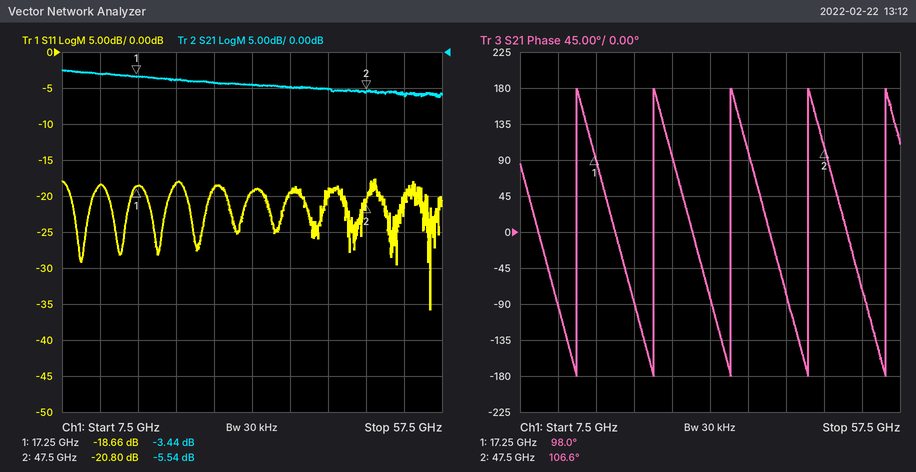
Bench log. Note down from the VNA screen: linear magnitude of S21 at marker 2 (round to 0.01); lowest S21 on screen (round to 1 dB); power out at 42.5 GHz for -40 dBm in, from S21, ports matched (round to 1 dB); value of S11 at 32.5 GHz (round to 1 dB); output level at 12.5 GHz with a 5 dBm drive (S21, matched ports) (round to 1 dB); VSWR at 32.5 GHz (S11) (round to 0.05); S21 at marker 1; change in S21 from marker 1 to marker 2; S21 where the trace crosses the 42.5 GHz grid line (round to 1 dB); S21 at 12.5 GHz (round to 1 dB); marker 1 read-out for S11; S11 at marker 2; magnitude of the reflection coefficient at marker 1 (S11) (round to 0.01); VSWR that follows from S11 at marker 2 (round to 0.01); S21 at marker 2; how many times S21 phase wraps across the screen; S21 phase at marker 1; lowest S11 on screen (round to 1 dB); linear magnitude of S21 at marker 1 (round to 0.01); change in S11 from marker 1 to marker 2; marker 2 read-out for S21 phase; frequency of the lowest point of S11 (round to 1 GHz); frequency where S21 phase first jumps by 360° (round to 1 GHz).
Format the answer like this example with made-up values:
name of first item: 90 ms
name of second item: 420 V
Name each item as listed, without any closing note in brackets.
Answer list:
linear magnitude of S21 at marker 2: 0.53
lowest S21 on screen: -6 dB
power out at 42.5 GHz for -40 dBm in, from S21, ports matched: -45 dBm
value of S11 at 32.5 GHz: -19 dB
output level at 12.5 GHz with a 5 dBm drive (S21, matched ports): 2 dBm
VSWR at 32.5 GHz (S11): 1.25
S21 at marker 1: -3.44 dB
change in S21 from marker 1 to marker 2: -2.10 dB
S21 where the trace crosses the 42.5 GHz grid line: -5 dB
S21 at 12.5 GHz: -3 dB
marker 1 read-out for S11: -18.66 dB
S11 at marker 2: -20.80 dB
magnitude of the reflection coefficient at marker 1 (S11): 0.12
VSWR that follows from S11 at marker 2: 1.20
S21 at marker 2: -5.54 dB
how many times S21 phase wraps across the screen: 5
S21 phase at marker 1: 98.0°
lowest S11 on screen: -36 dB
linear magnitude of S21 at marker 1: 0.67
change in S11 from marker 1 to marker 2: -2.14 dB
marker 2 read-out for S21 phase: 106.6°
frequency of the lowest point of S11: 56 GHz
frequency where S21 phase first jumps by 360°: 15 GHz
